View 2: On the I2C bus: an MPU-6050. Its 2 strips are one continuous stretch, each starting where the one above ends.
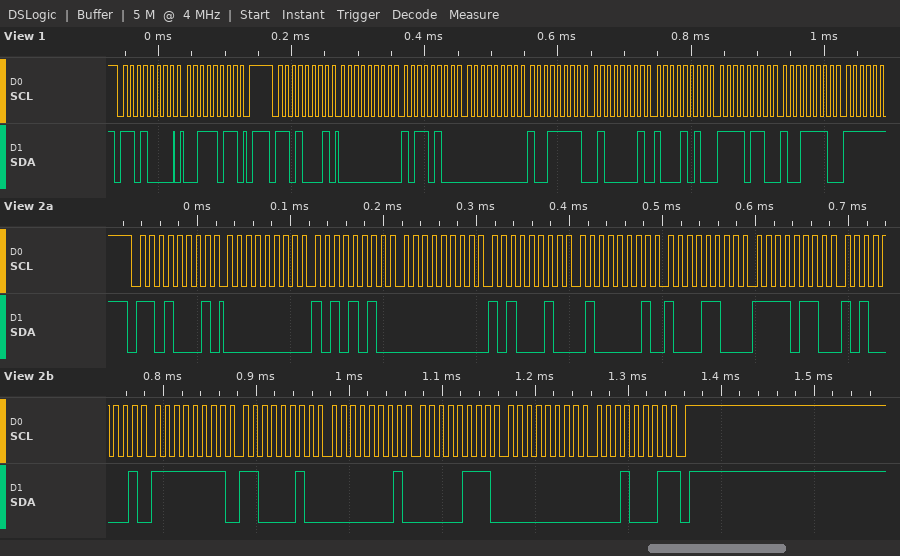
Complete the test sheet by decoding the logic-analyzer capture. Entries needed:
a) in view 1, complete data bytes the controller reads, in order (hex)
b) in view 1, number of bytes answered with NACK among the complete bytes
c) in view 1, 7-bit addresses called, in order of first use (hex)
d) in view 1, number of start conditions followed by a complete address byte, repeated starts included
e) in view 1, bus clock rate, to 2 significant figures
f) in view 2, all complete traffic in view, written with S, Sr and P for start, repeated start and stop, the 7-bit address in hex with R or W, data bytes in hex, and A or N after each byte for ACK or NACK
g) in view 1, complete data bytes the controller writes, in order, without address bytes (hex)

00 B4 00 9F 41 8A F6 9E
0
0x68
2
100 kHz
S 68R A 00 A AA A 00 A A2 A 41 A 8C A F6 A A1 A FF A C2 A 01 A 07 A 00 A 11 N P
3B
